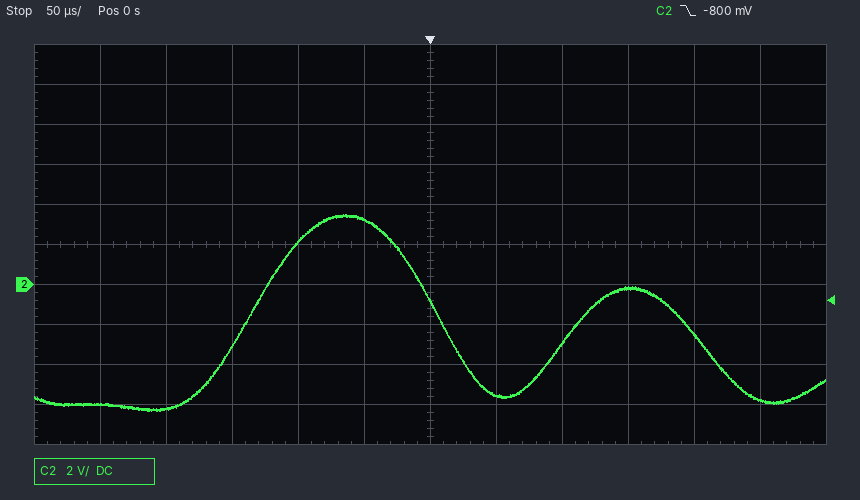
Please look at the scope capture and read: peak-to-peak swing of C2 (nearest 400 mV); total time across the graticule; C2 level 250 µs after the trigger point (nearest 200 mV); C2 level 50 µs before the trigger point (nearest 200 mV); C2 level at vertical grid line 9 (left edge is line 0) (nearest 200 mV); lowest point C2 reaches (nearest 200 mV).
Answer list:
10.0 V
600 µs
-5.8 V
3.2 V
-200 mV
-6.4 V
